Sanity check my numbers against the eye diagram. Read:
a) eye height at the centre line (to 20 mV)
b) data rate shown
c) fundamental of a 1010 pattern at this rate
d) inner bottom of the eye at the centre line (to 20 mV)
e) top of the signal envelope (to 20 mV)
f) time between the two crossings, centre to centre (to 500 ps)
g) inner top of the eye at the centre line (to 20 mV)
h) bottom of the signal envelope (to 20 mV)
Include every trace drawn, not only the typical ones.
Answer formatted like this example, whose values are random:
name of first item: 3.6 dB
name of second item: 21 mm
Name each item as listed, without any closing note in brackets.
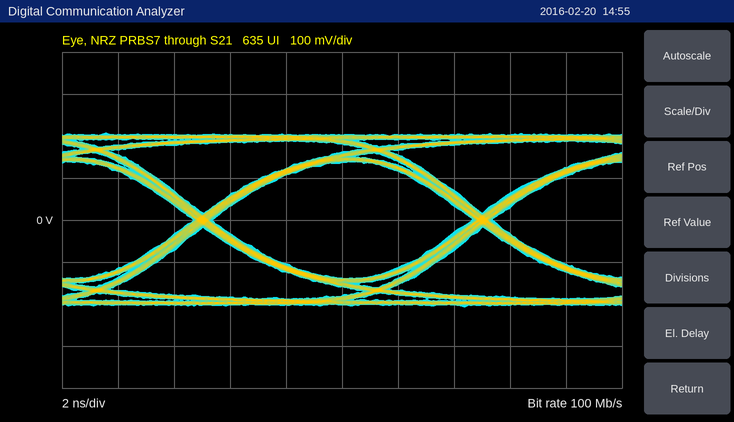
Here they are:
eye height at the centre line: 280 mV
data rate shown: 100 Mb/s
fundamental of a 1010 pattern at this rate: 50 MHz
inner bottom of the eye at the centre line: -140 mV
top of the signal envelope: 200 mV
time between the two crossings, centre to centre: 10.0 ns
inner top of the eye at the centre line: 140 mV
bottom of the signal envelope: -200 mV
